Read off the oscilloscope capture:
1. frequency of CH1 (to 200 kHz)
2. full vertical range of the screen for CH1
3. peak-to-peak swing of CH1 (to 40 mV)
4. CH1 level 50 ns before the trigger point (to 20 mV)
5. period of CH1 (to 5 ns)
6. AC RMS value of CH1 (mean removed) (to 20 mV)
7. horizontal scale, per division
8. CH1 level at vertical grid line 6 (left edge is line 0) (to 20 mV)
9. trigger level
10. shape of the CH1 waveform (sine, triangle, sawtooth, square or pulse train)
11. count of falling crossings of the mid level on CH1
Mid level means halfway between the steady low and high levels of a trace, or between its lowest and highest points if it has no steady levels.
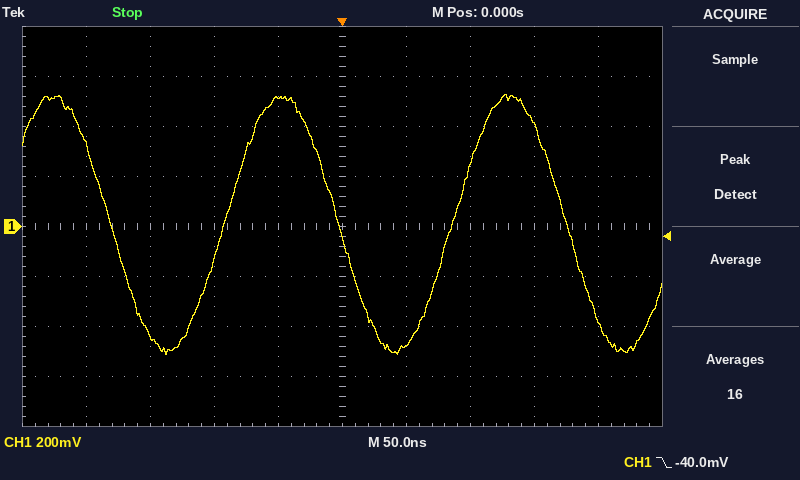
5.6 MHz
1.6 V
1.04 V
520 mV
180 ns
360 mV
50 ns
-480 mV
-40.0 mV
sine
3
